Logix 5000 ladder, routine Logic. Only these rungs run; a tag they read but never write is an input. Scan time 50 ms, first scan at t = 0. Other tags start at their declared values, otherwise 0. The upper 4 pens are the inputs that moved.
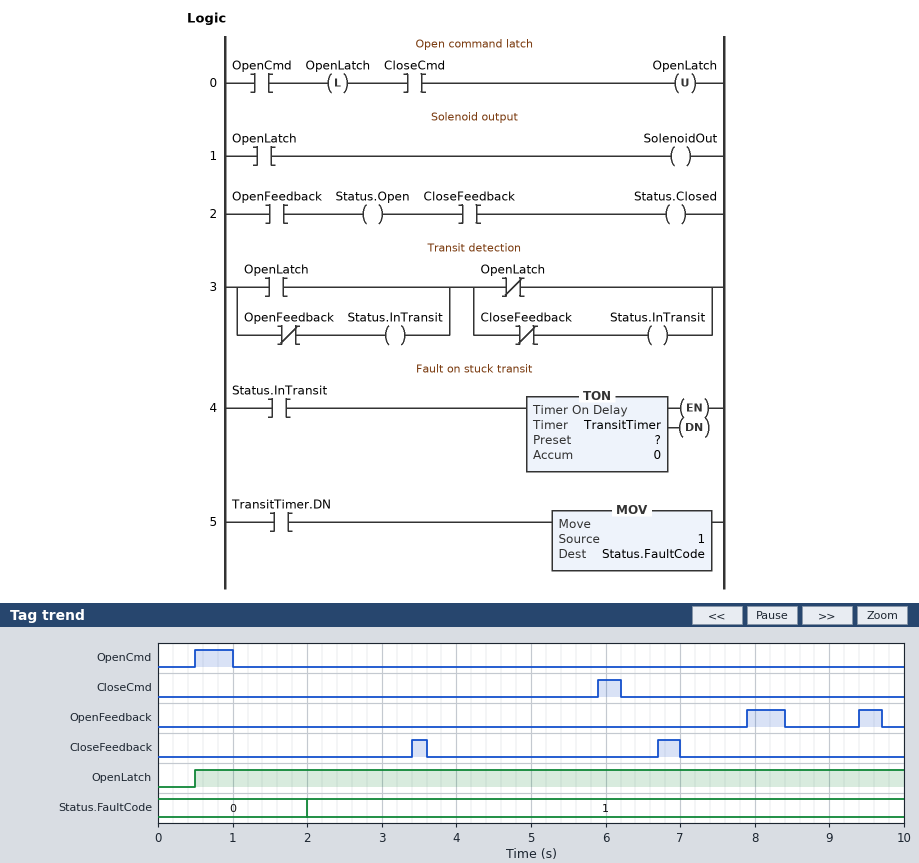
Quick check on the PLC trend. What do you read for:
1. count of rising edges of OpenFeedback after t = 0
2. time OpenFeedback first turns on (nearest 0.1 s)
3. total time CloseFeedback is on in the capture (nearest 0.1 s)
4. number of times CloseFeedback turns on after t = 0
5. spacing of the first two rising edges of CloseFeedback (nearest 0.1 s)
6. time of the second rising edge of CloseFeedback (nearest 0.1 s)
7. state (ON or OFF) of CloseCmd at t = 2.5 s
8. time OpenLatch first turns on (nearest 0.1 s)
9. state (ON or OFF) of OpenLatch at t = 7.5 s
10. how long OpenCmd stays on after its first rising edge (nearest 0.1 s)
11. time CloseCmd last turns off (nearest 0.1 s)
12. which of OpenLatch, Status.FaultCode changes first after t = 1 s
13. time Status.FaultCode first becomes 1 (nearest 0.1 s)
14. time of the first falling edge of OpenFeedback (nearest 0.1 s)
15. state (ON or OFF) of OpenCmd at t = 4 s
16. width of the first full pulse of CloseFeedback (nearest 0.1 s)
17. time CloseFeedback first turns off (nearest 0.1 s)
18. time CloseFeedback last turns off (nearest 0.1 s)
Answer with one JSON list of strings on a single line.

["2", "7.9 s", "0.5 s", "2", "3.3 s", "6.7 s", "OFF", "0.5 s", "ON", "0.5 s", "6.2 s", "Status.FaultCode", "2.0 s", "8.4 s", "OFF", "0.2 s", "3.6 s", "7.0 s"]
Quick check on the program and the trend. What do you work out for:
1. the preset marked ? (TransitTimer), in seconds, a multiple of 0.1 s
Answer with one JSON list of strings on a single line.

["2.0 s"]
